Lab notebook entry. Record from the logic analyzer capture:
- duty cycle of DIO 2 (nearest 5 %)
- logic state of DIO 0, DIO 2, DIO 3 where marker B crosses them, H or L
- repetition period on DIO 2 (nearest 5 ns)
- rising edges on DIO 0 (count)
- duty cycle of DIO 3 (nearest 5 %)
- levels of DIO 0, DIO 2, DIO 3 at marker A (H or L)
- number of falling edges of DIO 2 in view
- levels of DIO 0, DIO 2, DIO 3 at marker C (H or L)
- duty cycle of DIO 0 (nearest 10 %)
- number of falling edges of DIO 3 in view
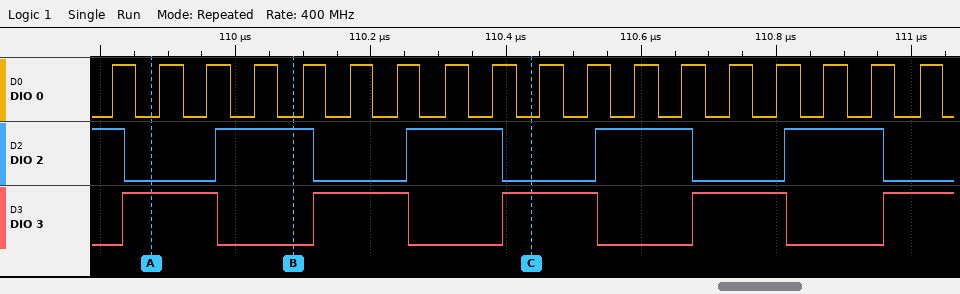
50 %
DIO 0=L, DIO 2=H, DIO 3=L
280 ns
18
50 %
DIO 0=L, DIO 2=L, DIO 3=H
5
DIO 0=L, DIO 2=L, DIO 3=H
50 %
4
